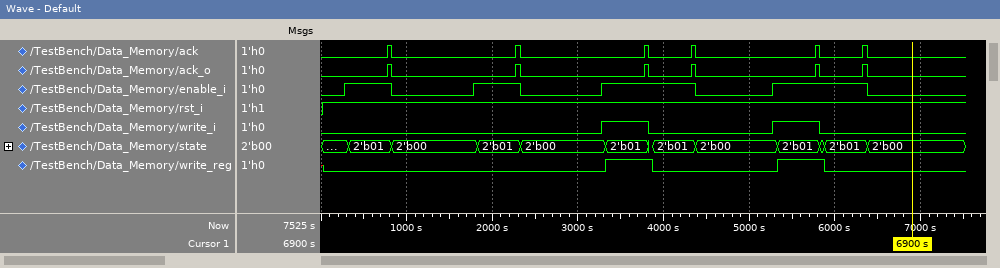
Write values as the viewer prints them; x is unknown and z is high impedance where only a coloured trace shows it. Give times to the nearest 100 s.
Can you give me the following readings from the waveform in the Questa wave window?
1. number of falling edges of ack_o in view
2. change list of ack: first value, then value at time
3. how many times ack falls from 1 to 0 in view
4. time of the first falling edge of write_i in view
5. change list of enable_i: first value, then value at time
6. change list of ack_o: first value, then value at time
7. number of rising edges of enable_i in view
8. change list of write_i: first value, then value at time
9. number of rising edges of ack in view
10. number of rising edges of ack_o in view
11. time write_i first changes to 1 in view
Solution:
6
0, 1 at 800 s, 0 at 800 s, 1 at 2300 s, 0 at 2300 s, 1 at 3800 s, 0 at 3800 s, 1 at 4300 s, 0 at 4400 s, 1 at 5800 s, 0 at 5800 s, 1 at 6300 s, 0 at 6400 s
6
3800 s
0, 1 at 300 s, 0 at 800 s, 1 at 1800 s, 0 at 2300 s, 1 at 3300 s, 0 at 4400 s, 1 at 5300 s, 0 at 6400 s
0, 1 at 800 s, 0 at 800 s, 1 at 2300 s, 0 at 2300 s, 1 at 3800 s, 0 at 3800 s, 1 at 4300 s, 0 at 4400 s, 1 at 5800 s, 0 at 5800 s, 1 at 6300 s, 0 at 6400 s
4
0, 1 at 3300 s, 0 at 3800 s, 1 at 5300 s, 0 at 5800 s
6
6
3300 s
